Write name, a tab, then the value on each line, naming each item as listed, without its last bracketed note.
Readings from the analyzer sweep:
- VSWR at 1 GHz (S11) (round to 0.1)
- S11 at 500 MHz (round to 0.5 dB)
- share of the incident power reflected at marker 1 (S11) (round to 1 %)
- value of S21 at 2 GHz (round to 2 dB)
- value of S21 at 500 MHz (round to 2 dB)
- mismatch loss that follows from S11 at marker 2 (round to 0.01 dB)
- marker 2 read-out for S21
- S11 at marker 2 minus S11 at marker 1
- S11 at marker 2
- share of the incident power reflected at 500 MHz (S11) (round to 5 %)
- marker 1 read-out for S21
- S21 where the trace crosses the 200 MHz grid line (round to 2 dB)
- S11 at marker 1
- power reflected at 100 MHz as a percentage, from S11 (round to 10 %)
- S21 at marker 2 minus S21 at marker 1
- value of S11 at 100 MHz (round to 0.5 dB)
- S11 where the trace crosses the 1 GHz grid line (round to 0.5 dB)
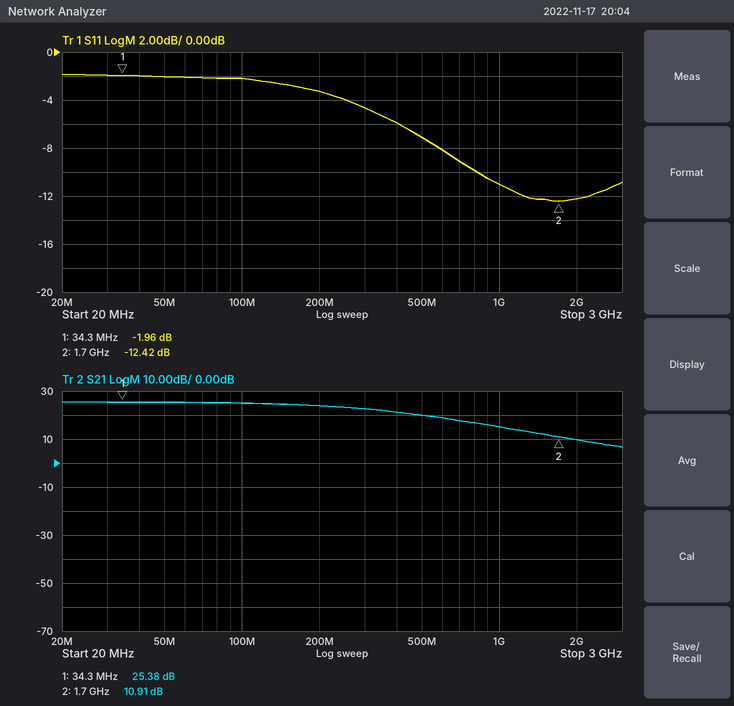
VSWR at 1 GHz (S11)	1.8
S11 at 500 MHz	-7.0 dB
share of the incident power reflected at marker 1 (S11)	64 %
value of S21 at 2 GHz	10 dB
value of S21 at 500 MHz	20 dB
mismatch loss that follows from S11 at marker 2	0.26 dB
marker 2 read-out for S21	10.91 dB
S11 at marker 2 minus S11 at marker 1	-10.46 dB
S11 at marker 2	-12.42 dB
share of the incident power reflected at 500 MHz (S11)	20 %
marker 1 read-out for S21	25.38 dB
S21 where the trace crosses the 200 MHz grid line	24 dB
S11 at marker 1	-1.96 dB
power reflected at 100 MHz as a percentage, from S11	60 %
S21 at marker 2 minus S21 at marker 1	-14.47 dB
value of S11 at 100 MHz	-2.0 dB
S11 where the trace crosses the 1 GHz grid line	-11.0 dB
